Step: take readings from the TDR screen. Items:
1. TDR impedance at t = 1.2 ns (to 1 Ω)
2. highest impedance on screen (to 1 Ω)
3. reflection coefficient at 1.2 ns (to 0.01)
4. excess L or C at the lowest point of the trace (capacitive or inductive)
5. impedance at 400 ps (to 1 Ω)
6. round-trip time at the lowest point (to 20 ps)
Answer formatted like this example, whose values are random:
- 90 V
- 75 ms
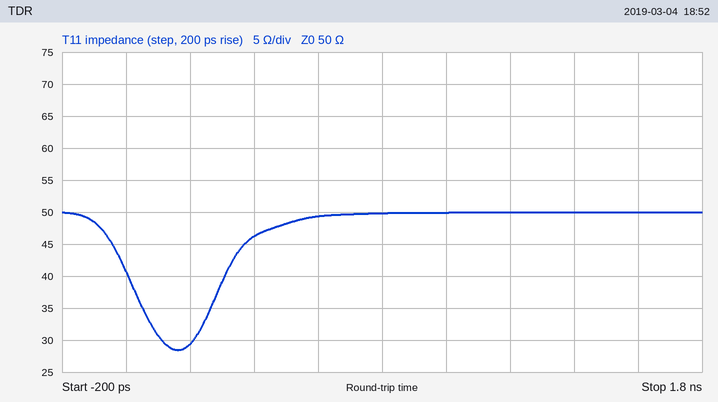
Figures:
- 50 Ω
- 50 Ω
- 0.00
- capacitive
- 46 Ω
- 160 ps
